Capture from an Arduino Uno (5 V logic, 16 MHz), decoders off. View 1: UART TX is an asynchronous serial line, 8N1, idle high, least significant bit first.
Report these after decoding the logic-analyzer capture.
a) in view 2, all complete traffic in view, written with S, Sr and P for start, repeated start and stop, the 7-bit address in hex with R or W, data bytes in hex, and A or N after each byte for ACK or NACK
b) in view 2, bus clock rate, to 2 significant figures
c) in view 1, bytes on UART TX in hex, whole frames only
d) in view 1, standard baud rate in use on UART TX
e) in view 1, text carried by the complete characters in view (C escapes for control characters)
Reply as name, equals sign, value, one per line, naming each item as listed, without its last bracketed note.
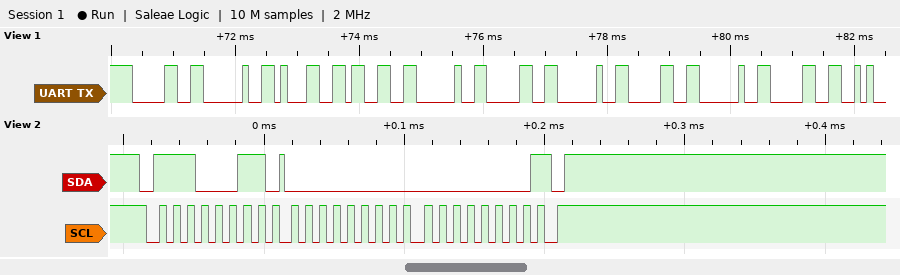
in view 2, all complete traffic in view, written with S, Sr and P for start, repeated start and stop, the 7-bit address in hex with R or W, data bytes in hex, and A or N after each byte for ACK or NACK = S 71R A 00 A 00 N P
in view 2, bus clock rate, to 2 significant figures = 100 kHz
in view 1, bytes on UART TX in hex, whole frames only = 30 20 31 33 20 30 20 30 20 30
in view 1, standard baud rate in use on UART TX = 9600 baud
in view 1, text carried by the complete characters in view = "0 13 0 0 0"
